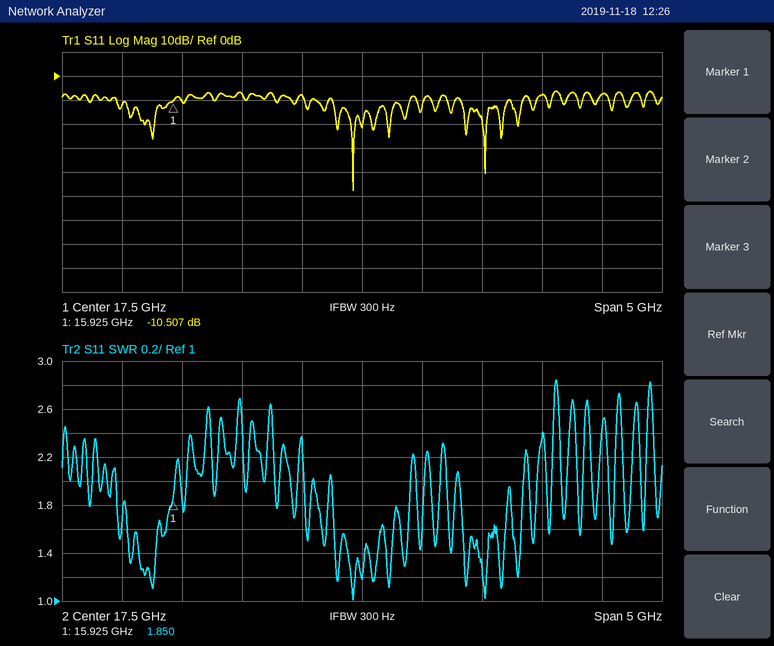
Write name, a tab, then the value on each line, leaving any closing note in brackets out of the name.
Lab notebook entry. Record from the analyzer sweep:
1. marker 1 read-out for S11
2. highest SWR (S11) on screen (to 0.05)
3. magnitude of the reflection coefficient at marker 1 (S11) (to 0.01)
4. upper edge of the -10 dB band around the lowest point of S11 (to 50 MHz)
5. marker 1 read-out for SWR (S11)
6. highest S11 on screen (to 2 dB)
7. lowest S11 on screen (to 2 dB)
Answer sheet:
marker 1 read-out for S11	-10.507 dB
highest SWR (S11) on screen	2.85
magnitude of the reflection coefficient at marker 1 (S11)	0.30
upper edge of the -10 dB band around the lowest point of S11	17.90 GHz
marker 1 read-out for SWR	1.850
highest S11 on screen	-6 dB
lowest S11 on screen	-48 dB
